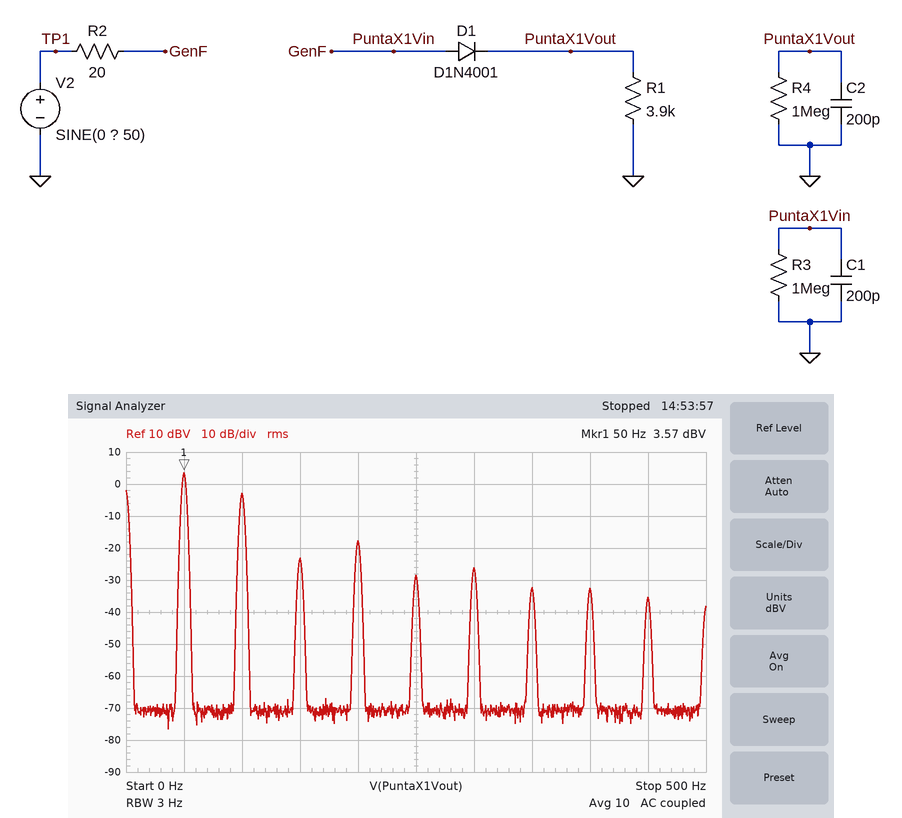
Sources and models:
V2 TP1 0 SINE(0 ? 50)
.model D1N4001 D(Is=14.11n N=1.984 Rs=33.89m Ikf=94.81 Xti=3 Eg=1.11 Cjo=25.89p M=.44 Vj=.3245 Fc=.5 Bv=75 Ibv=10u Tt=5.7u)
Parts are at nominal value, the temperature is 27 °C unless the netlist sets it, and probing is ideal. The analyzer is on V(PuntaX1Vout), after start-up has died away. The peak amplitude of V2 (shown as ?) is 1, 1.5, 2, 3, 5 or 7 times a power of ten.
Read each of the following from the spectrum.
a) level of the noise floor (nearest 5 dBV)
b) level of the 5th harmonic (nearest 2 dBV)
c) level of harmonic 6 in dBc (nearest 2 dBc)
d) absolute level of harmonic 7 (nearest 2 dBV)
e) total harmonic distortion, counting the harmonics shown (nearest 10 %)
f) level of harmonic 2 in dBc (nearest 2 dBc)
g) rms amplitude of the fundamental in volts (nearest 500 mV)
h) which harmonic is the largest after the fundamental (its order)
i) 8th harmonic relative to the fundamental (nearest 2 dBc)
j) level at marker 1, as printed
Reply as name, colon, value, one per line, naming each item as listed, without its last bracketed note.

level of the noise floor: -70 dBV
level of the 5th harmonic: -28 dBV
level of harmonic 6 in dBc: -30 dBc
absolute level of harmonic 7: -32 dBV
total harmonic distortion, counting the harmonics shown: 50 %
level of harmonic 2 in dBc: -6 dBc
rms amplitude of the fundamental in volts: 1.5 V
which harmonic is the largest after the fundamental: 2
8th harmonic relative to the fundamental: -36 dBc
level at marker 1, as printed: 3.57 dBV
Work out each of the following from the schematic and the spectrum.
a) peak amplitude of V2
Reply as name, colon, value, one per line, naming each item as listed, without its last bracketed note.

peak amplitude of V2: 5 V
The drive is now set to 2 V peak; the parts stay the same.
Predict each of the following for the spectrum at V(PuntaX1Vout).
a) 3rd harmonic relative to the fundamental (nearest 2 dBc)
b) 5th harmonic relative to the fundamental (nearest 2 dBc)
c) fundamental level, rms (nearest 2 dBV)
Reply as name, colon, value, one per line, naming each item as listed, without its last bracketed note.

3rd harmonic relative to the fundamental: -18 dBc
5th harmonic relative to the fundamental: -26 dBc
fundamental level, rms: -6 dBV
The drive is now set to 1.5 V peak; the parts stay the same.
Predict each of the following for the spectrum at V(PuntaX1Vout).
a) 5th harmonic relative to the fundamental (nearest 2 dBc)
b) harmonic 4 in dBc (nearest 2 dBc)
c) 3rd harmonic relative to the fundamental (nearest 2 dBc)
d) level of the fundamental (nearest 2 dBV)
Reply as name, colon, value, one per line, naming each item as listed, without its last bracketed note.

5th harmonic relative to the fundamental: -24 dBc
harmonic 4 in dBc: -26 dBc
3rd harmonic relative to the fundamental: -16 dBc
level of the fundamental: -10 dBV
